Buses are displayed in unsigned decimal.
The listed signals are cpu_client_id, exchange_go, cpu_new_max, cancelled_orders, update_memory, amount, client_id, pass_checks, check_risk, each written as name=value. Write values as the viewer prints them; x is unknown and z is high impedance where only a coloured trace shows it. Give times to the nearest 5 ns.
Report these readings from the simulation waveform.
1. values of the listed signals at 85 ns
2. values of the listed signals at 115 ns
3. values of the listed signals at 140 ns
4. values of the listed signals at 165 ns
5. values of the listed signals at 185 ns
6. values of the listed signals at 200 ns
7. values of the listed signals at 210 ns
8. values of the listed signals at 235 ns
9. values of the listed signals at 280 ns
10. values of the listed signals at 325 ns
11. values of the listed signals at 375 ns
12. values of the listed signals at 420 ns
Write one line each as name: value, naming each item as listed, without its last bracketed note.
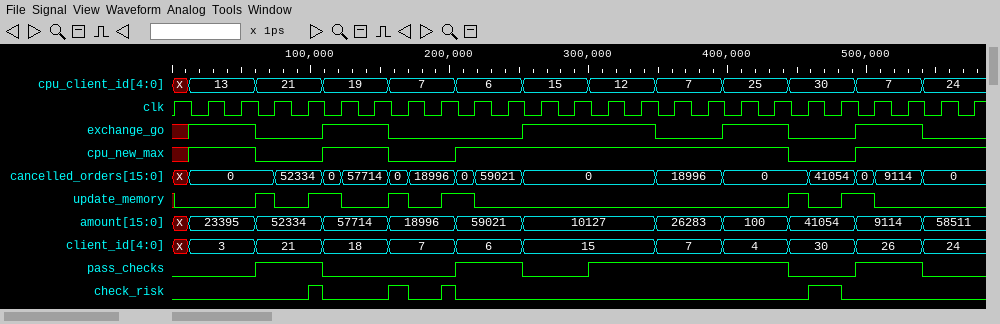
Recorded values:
values of the listed signals at 85 ns: cpu_client_id=21, exchange_go=0, cpu_new_max=0, cancelled_orders=52334, update_memory=0, amount=52334, client_id=21, pass_checks=1, check_risk=0
values of the listed signals at 115 ns: cpu_client_id=19, exchange_go=1, cpu_new_max=1, cancelled_orders=0, update_memory=1, amount=57714, client_id=18, pass_checks=0, check_risk=0
values of the listed signals at 140 ns: cpu_client_id=19, exchange_go=1, cpu_new_max=1, cancelled_orders=57714, update_memory=0, amount=57714, client_id=18, pass_checks=0, check_risk=0
values of the listed signals at 165 ns: cpu_client_id=7, exchange_go=0, cpu_new_max=0, cancelled_orders=0, update_memory=1, amount=18996, client_id=7, pass_checks=0, check_risk=1
values of the listed signals at 185 ns: cpu_client_id=7, exchange_go=0, cpu_new_max=0, cancelled_orders=18996, update_memory=0, amount=18996, client_id=7, pass_checks=0, check_risk=0
values of the listed signals at 200 ns: cpu_client_id=7, exchange_go=0, cpu_new_max=0, cancelled_orders=18996, update_memory=1, amount=18996, client_id=7, pass_checks=0, check_risk=1
values of the listed signals at 210 ns: cpu_client_id=6, exchange_go=0, cpu_new_max=1, cancelled_orders=0, update_memory=1, amount=59021, client_id=6, pass_checks=1, check_risk=0
values of the listed signals at 235 ns: cpu_client_id=6, exchange_go=0, cpu_new_max=1, cancelled_orders=59021, update_memory=0, amount=59021, client_id=6, pass_checks=1, check_risk=0
values of the listed signals at 280 ns: cpu_client_id=15, exchange_go=1, cpu_new_max=1, cancelled_orders=0, update_memory=0, amount=10127, client_id=15, pass_checks=0, check_risk=0
values of the listed signals at 325 ns: cpu_client_id=12, exchange_go=1, cpu_new_max=1, cancelled_orders=0, update_memory=0, amount=10127, client_id=15, pass_checks=1, check_risk=0
values of the listed signals at 375 ns: cpu_client_id=7, exchange_go=0, cpu_new_max=1, cancelled_orders=18996, update_memory=0, amount=26283, client_id=7, pass_checks=1, check_risk=0
values of the listed signals at 420 ns: cpu_client_id=25, exchange_go=1, cpu_new_max=1, cancelled_orders=0, update_memory=0, amount=100, client_id=4, pass_checks=1, check_risk=0
